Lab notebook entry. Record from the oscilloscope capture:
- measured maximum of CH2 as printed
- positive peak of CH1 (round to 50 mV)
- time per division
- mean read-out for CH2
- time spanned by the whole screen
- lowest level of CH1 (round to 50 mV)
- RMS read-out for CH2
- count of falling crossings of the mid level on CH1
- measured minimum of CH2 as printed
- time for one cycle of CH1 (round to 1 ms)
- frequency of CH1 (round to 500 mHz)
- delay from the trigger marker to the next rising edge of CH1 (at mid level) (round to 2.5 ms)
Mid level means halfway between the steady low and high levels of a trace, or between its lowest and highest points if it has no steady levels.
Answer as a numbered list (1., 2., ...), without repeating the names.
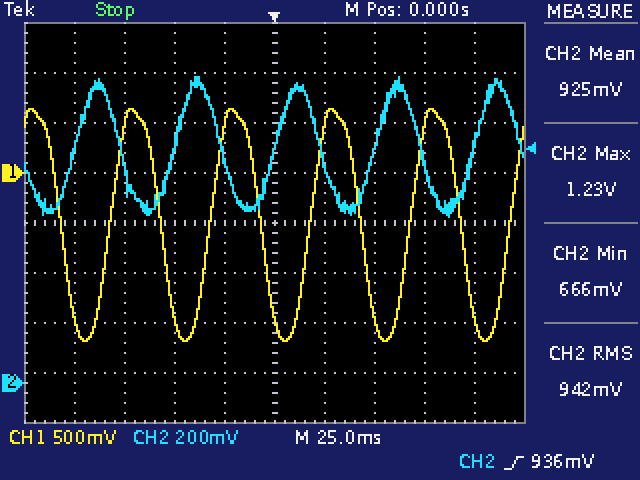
1. 1.23 V
2. 650 mV
3. 25 ms
4. 925 mV
5. 250 ms
6. -1.70 V
7. 942 mV
8. 5
9. 666 mV
10. 50 ms
11. 20.0 Hz
12. 17.5 ms
